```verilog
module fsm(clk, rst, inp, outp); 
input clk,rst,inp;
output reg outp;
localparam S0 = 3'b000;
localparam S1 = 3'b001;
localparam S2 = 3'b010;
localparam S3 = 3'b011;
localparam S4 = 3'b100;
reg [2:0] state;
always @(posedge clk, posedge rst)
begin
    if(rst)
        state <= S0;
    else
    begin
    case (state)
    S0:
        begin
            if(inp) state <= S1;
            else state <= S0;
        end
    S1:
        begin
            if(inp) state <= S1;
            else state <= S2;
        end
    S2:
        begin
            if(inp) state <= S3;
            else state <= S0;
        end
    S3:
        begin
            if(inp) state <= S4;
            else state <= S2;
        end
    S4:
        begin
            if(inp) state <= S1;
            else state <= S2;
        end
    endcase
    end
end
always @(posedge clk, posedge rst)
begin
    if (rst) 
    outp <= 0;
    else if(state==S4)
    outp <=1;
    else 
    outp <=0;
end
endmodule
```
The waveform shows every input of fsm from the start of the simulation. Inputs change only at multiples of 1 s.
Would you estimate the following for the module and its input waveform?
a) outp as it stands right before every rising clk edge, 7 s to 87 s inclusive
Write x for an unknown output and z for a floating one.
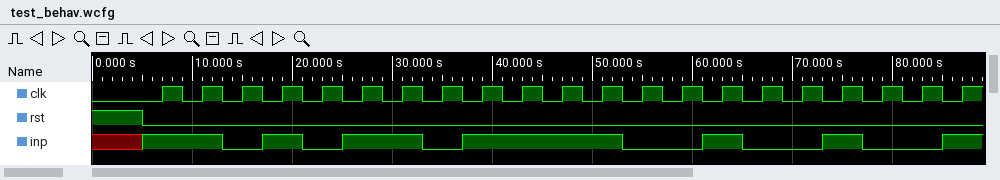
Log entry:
0 0 0 0 0 0 0 0 1 0 0 1 0 0 0 0 0 0 0 0 0
